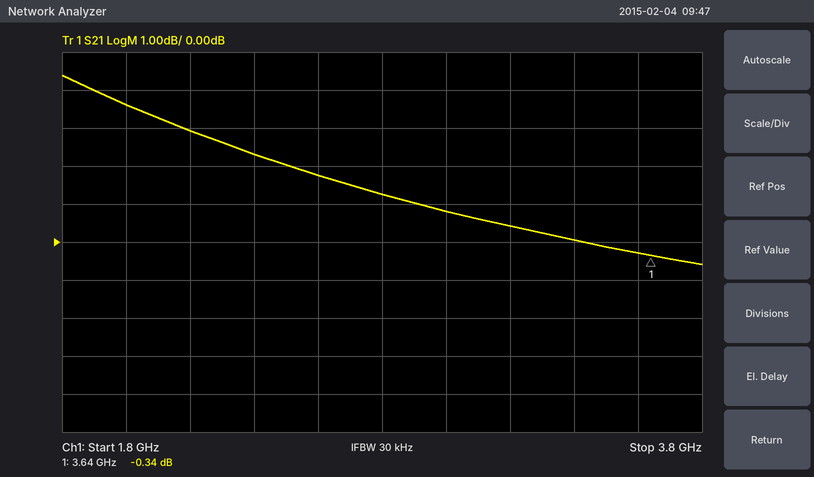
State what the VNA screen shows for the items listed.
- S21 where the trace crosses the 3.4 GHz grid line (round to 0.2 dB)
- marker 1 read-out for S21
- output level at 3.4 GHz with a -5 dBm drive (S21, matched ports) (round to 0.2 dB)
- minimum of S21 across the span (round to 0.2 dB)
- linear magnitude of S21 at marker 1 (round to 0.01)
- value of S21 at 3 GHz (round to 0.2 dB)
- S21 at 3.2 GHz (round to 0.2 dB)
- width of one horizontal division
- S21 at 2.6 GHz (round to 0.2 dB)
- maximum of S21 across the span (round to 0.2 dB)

0.0 dB
-0.34 dB
-5.0 dBm
-0.6 dB
0.96
0.8 dB
0.4 dB
200 MHz
1.8 dB
4.4 dB
